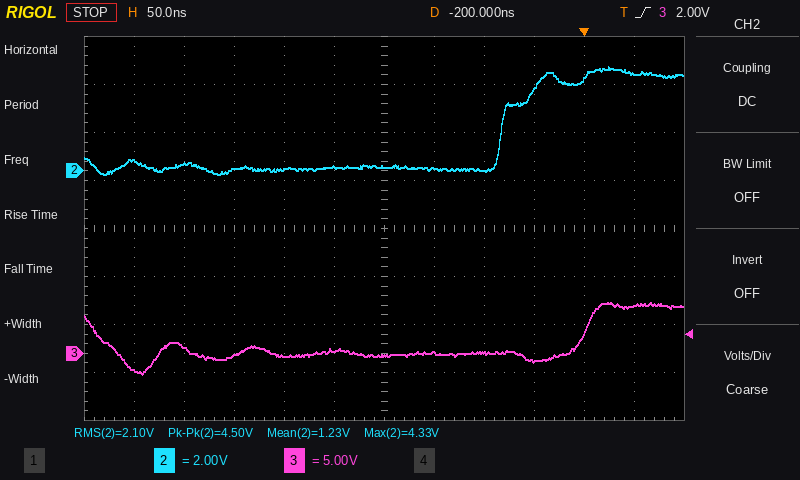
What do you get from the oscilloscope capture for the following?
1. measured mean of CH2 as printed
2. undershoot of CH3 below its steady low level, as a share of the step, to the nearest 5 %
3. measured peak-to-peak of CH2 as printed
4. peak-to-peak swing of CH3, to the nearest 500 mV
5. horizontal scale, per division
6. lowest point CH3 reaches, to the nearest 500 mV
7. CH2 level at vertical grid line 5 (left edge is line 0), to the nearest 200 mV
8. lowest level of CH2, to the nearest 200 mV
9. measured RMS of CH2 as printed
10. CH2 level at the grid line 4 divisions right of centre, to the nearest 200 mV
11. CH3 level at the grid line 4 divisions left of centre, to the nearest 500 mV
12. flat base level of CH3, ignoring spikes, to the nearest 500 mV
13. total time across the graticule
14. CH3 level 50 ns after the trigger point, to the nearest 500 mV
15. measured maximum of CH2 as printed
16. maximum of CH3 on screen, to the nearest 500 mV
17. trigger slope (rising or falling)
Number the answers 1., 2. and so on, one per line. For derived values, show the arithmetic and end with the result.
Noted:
1. 1.23 V
2. 40 %
3. 4.50 V
4. 5.5 V − (-2.0 V) = 7.5 V
5. 50 ns
6. -2.0 V
7. 200 mV
8. -200 mV
9. 2.10 V
10. 3.8 V
11. 500 mV
12. 0.0 V
13. 600 ns
14. 5.0 V
15. 4.33 V
16. 5.5 V
17. rising
